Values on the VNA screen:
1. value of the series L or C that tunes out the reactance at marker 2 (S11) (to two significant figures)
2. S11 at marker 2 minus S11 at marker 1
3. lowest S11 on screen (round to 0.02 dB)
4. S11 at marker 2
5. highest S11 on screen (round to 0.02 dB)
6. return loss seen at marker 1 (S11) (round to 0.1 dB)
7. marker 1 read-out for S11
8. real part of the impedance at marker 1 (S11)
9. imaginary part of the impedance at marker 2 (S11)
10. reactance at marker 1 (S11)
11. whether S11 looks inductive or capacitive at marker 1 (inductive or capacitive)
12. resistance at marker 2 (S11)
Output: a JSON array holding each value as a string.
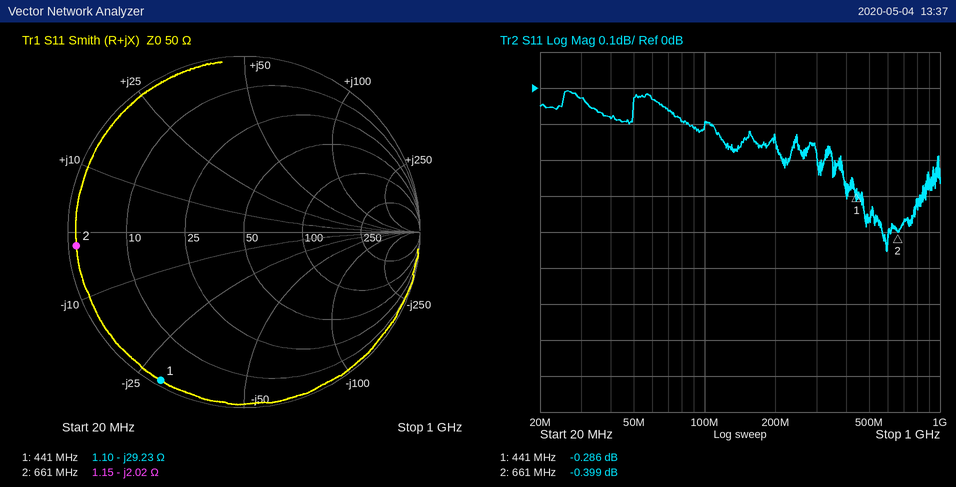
["490 pH", "-0.113 dB", "-0.46 dB", "-0.399 dB", "0.00 dB", "0.3 dB", "-0.286 dB", "1.10 Ω", "-2.02 Ω", "-29.23 Ω", "capacitive", "1.15 Ω"]
